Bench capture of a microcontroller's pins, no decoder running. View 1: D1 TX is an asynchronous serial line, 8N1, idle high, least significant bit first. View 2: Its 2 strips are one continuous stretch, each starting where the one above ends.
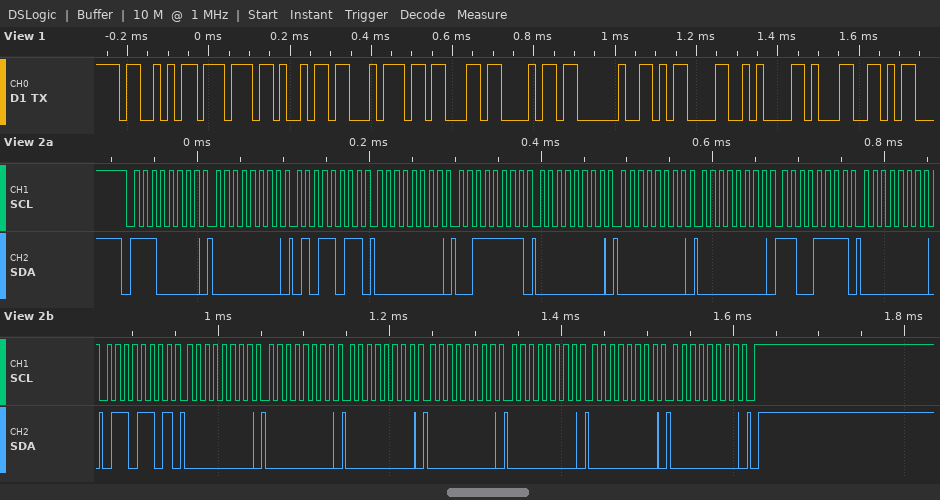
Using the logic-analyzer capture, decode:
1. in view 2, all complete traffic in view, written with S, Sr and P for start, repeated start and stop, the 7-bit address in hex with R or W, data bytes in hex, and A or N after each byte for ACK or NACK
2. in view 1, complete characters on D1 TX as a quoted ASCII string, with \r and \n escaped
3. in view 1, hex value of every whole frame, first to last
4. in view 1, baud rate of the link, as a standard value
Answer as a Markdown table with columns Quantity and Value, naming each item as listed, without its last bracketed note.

| Quantity | Value |
|---|---|
| in view 2, all complete traffic in view, written with S, Sr and P for start, repeated start and stop, the 7-bit address in hex with R or W, data bytes in hex, and A or N after each byte for ACK or NACK | S 70W A 00 A 5B A 00 A 3F A 00 A 00 A 00 A CF A 00 A 6D A 00 A 00 A 00 A 00 A 00 A 00 A 00 A P |
| in view 1, complete characters on D1 TX as a quoted ASCII string, with \r and \n escaped | "Switch \r\n1" |
| in view 1, hex value of every whole frame, first to last | 53 77 69 74 63 68 20 0D 0A 31 |
| in view 1, baud rate of the link, as a standard value | 57600 baud |
